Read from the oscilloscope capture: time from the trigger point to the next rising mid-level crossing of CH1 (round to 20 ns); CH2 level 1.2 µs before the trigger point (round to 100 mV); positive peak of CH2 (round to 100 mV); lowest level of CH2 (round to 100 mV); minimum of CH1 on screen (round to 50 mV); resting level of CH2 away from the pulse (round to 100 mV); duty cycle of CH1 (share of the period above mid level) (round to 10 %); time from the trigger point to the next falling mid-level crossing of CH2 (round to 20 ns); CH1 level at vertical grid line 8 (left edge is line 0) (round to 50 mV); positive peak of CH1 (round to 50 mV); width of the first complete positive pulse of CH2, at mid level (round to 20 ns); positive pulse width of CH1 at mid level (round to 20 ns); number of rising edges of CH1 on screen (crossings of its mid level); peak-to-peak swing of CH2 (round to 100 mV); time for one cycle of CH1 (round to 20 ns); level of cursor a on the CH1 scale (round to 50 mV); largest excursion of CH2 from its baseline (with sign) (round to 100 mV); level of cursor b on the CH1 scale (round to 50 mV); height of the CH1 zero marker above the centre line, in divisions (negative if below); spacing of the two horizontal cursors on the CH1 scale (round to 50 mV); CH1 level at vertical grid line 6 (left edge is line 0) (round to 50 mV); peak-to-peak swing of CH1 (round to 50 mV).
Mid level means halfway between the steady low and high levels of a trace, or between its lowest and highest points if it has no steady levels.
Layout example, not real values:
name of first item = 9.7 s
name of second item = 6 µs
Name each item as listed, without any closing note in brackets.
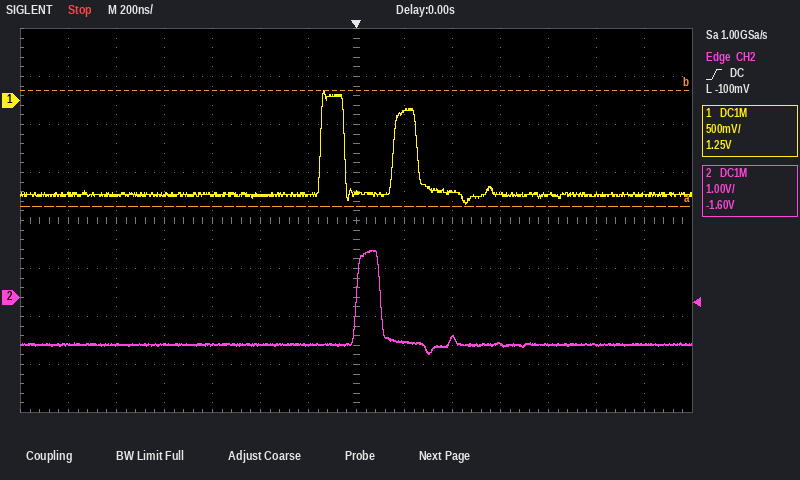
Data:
time from the trigger point to the next rising mid-level crossing of CH1 = 160 ns
CH2 level 1.2 µs before the trigger point = -1.0 V
positive peak of CH2 = 1.0 V
lowest level of CH2 = -1.2 V
minimum of CH1 on screen = -1.10 V
resting level of CH2 away from the pulse = -1.0 V
duty cycle of CH1 (share of the period above mid level) = 30 %
time from the trigger point to the next falling mid-level crossing of CH2 = 100 ns
CH1 level at vertical grid line 8 (left edge is line 0) = -100 mV
positive peak of CH1 = 100 mV
width of the first complete positive pulse of CH2, at mid level = 100 ns
positive pulse width of CH1 at mid level = 100 ns
number of rising edges of CH1 on screen = 2
peak-to-peak swing of CH2 = 2.2 V
time for one cycle of CH1 = 300 ns
level of cursor a on the CH1 scale = -1.10 V
largest excursion of CH2 from its baseline (with sign) = +2.0 V
level of cursor b on the CH1 scale = 100 mV
height of the CH1 zero marker above the centre line, in divisions = +2.5 div
spacing of the two horizontal cursors on the CH1 scale = 1.20 V
CH1 level at vertical grid line 6 (left edge is line 0) = -1.00 V
peak-to-peak swing of CH1 = 1.20 V
